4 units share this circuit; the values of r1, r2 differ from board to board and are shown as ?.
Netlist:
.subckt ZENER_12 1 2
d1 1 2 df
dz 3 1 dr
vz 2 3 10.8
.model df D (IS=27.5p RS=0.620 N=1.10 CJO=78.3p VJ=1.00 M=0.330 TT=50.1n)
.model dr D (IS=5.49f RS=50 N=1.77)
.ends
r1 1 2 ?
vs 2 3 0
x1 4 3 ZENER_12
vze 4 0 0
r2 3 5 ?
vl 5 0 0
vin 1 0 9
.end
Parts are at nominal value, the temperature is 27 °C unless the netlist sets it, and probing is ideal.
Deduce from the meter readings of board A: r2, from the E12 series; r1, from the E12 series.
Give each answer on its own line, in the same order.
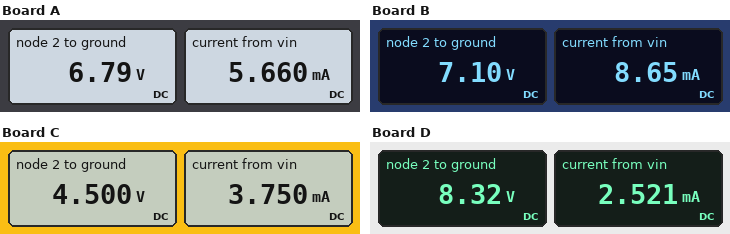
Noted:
1.2 kΩ
390 Ω
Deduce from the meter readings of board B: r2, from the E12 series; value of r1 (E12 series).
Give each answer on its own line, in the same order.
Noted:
820 Ω
220 Ω
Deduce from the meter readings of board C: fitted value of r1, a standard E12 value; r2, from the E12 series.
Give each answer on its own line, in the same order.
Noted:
1.2 kΩ
1.2 kΩ
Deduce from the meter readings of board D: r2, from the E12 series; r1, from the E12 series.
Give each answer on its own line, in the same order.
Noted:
3.3 kΩ
270 Ω
